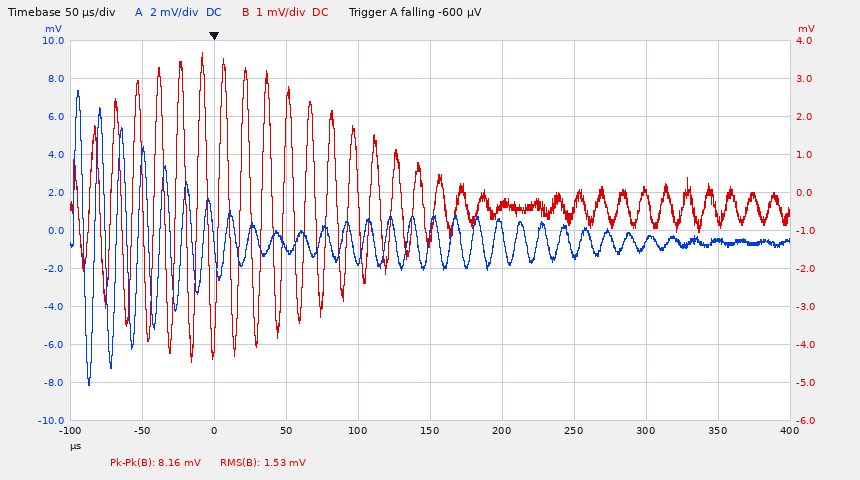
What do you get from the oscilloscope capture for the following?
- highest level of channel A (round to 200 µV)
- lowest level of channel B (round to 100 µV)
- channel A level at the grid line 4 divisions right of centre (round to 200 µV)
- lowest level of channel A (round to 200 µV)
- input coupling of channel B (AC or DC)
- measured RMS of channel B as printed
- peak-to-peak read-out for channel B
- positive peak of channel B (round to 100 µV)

7.4 mV
-4.5 mV
-600 µV
-8.2 mV
DC
1.53 mV
8.16 mV
3.7 mV
